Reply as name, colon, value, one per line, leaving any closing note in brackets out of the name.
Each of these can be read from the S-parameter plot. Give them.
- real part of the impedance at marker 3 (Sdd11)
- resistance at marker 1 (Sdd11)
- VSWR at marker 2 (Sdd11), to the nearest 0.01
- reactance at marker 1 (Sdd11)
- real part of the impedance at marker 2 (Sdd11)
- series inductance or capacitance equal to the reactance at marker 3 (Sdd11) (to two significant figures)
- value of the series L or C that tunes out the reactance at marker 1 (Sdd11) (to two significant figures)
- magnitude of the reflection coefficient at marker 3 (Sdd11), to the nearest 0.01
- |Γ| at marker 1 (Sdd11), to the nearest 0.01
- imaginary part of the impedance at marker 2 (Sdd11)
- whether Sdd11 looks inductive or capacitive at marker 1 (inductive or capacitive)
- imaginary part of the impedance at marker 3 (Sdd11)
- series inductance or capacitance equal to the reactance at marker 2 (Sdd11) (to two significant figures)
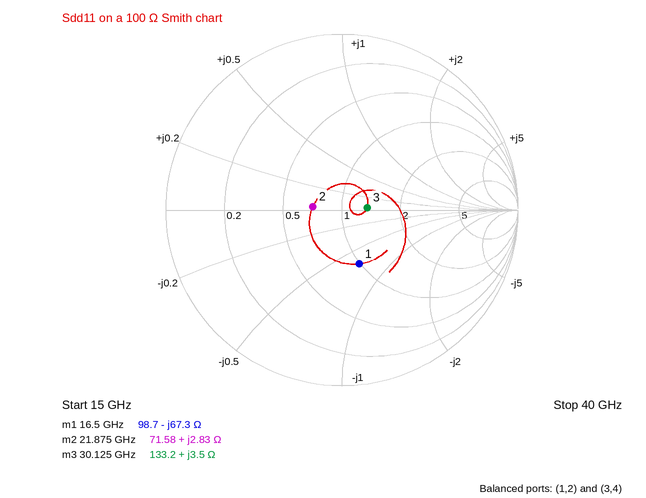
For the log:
real part of the impedance at marker 3: 133.2 Ω
resistance at marker 1: 98.7 Ω
VSWR at marker 2 (Sdd11), to the nearest 0.01: 1.40
reactance at marker 1: -67.3 Ω
real part of the impedance at marker 2: 71.58 Ω
series inductance or capacitance equal to the reactance at marker 3 (Sdd11): 18 pH
value of the series L or C that tunes out the reactance at marker 1 (Sdd11): 650 pH
magnitude of the reflection coefficient at marker 3 (Sdd11), to the nearest 0.01: 0.14
|Γ| at marker 1 (Sdd11), to the nearest 0.01: 0.32
imaginary part of the impedance at marker 2: +2.83 Ω
whether Sdd11 looks inductive or capacitive at marker 1: capacitive
imaginary part of the impedance at marker 3: +3.5 Ω
series inductance or capacitance equal to the reactance at marker 2 (Sdd11): 21 pH
